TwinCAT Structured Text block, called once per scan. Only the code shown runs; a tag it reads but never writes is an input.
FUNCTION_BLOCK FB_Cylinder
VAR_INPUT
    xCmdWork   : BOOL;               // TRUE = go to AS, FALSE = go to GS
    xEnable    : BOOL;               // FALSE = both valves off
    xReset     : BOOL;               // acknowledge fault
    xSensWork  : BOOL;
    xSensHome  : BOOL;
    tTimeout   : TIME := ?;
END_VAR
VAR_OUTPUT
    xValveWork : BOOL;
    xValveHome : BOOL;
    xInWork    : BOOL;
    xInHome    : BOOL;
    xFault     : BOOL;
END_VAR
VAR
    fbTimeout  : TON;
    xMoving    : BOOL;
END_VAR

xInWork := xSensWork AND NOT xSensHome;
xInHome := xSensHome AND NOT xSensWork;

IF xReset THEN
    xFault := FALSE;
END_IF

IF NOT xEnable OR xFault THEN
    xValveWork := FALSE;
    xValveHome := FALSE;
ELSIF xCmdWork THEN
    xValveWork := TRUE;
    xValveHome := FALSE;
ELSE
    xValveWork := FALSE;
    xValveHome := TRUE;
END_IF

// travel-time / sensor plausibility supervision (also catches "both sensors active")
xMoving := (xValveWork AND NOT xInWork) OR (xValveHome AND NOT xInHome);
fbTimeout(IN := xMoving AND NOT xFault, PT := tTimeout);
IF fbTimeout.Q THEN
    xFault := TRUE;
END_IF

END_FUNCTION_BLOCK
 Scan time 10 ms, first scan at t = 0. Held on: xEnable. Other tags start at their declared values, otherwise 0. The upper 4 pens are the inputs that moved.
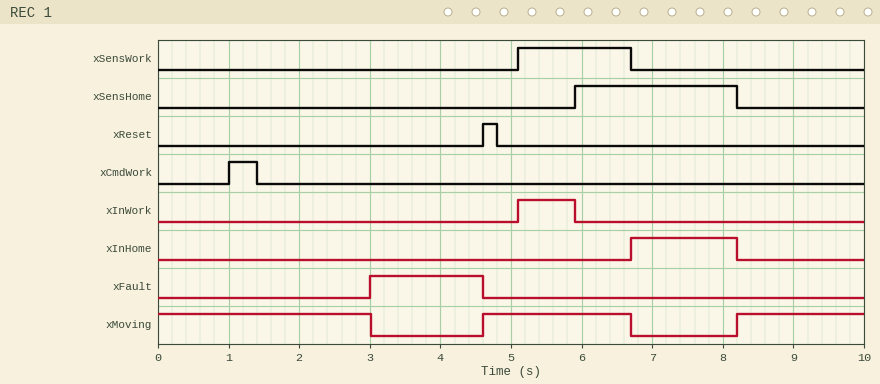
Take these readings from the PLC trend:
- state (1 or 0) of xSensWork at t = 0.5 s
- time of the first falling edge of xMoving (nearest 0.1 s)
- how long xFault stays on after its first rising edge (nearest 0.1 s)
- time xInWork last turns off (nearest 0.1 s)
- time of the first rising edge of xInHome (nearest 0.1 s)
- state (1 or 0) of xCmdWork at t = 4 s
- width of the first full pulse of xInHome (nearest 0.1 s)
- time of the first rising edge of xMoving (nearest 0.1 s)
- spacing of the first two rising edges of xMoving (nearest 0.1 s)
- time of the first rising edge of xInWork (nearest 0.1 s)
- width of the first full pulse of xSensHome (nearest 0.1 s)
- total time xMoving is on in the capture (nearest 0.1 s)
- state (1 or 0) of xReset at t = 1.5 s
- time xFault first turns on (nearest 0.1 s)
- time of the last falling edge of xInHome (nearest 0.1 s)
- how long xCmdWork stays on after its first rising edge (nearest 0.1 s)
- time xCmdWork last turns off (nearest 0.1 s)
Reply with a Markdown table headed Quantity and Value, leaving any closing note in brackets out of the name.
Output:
| Quantity | Value |
|---|---|
| state (1 or 0) of xSensWork at t = 0.5 s | 0 |
| time of the first falling edge of xMoving | 3.0 s |
| how long xFault stays on after its first rising edge | 1.6 s |
| time xInWork last turns off | 5.9 s |
| time of the first rising edge of xInHome | 6.7 s |
| state (1 or 0) of xCmdWork at t = 4 s | 0 |
| width of the first full pulse of xInHome | 1.5 s |
| time of the first rising edge of xMoving | 4.6 s |
| spacing of the first two rising edges of xMoving | 3.6 s |
| time of the first rising edge of xInWork | 5.1 s |
| width of the first full pulse of xSensHome | 2.3 s |
| total time xMoving is on in the capture | 6.9 s |
| state (1 or 0) of xReset at t = 1.5 s | 0 |
| time xFault first turns on | 3.0 s |
| time of the last falling edge of xInHome | 8.2 s |
| how long xCmdWork stays on after its first rising edge | 0.4 s |
| time xCmdWork last turns off | 1.4 s |
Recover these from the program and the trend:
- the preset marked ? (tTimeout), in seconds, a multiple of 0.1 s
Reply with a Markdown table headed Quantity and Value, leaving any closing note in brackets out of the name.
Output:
| Quantity | Value |
|---|---|
| the preset marked ? (tTimeout), in seconds, a multiple of 0.1 s | 3.0 s |
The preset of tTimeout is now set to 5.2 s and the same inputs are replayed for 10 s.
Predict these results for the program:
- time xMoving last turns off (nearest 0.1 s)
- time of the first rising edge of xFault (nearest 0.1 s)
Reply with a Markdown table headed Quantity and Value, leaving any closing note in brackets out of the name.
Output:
| Quantity | Value |
|---|---|
| time xMoving last turns off | 5.2 s |
| time of the first rising edge of xFault | 5.2 s |
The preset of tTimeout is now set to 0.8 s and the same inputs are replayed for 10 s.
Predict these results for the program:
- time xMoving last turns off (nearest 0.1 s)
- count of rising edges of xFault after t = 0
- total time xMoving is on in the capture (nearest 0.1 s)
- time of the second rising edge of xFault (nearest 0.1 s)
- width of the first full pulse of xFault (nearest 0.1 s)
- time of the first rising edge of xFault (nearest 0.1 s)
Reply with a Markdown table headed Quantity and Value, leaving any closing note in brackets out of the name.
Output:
| Quantity | Value |
|---|---|
| time xMoving last turns off | 5.4 s |
| count of rising edges of xFault after t = 0 | 2 |
| total time xMoving is on in the capture | 1.6 s |
| time of the second rising edge of xFault | 5.4 s |
| width of the first full pulse of xFault | 3.8 s |
| time of the first rising edge of xFault | 0.8 s |
